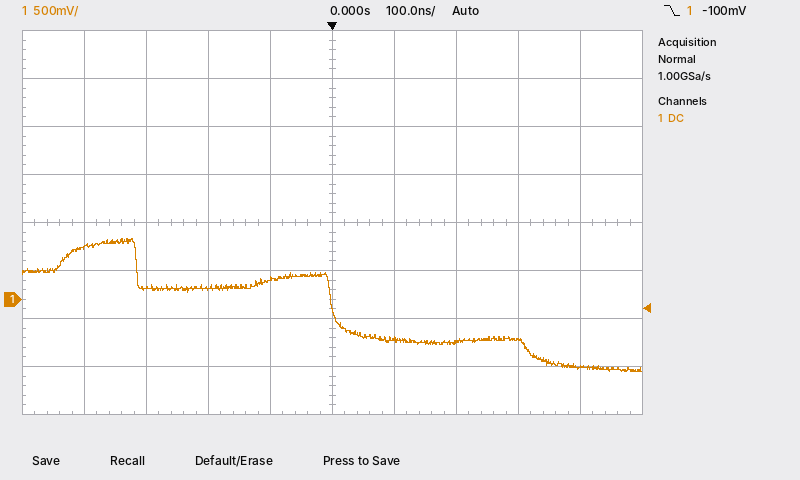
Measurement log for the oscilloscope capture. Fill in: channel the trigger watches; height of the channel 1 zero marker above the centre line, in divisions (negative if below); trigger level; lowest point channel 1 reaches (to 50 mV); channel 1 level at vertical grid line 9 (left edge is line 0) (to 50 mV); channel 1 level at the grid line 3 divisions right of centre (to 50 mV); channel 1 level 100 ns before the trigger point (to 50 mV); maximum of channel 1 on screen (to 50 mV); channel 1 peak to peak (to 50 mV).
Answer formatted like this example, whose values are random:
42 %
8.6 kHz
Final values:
channel 1
-1.6 div
-100 mV
-750 mV
-700 mV
-400 mV
200 mV
650 mV
1.40 V
